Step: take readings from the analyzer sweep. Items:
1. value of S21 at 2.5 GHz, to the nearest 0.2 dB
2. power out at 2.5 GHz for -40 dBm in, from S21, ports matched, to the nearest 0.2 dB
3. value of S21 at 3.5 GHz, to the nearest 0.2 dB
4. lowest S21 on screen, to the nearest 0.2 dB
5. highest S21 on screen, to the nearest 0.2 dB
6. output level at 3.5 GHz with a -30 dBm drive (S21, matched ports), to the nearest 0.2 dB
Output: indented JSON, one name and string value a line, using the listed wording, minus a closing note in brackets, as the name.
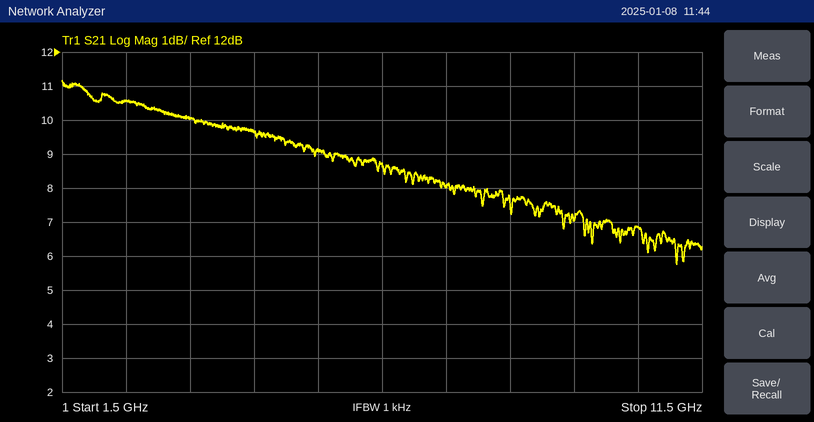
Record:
{
  "value of S21 at 2.5 GHz, to the nearest 0.2 dB": "10.6 dB",
  "power out at 2.5 GHz for -40 dBm in, from S21, ports matched, to the nearest 0.2 dB": "-29.4 dBm",
  "value of S21 at 3.5 GHz, to the nearest 0.2 dB": "10.0 dB",
  "lowest S21 on screen, to the nearest 0.2 dB": "5.8 dB",
  "highest S21 on screen, to the nearest 0.2 dB": "11.2 dB",
  "output level at 3.5 GHz with a -30 dBm drive (S21, matched ports), to the nearest 0.2 dB": "-20.0 dBm"
}
